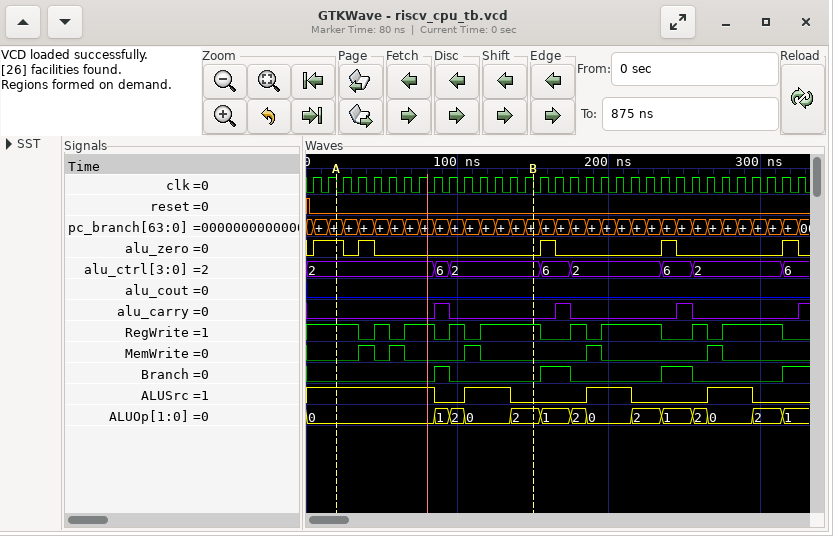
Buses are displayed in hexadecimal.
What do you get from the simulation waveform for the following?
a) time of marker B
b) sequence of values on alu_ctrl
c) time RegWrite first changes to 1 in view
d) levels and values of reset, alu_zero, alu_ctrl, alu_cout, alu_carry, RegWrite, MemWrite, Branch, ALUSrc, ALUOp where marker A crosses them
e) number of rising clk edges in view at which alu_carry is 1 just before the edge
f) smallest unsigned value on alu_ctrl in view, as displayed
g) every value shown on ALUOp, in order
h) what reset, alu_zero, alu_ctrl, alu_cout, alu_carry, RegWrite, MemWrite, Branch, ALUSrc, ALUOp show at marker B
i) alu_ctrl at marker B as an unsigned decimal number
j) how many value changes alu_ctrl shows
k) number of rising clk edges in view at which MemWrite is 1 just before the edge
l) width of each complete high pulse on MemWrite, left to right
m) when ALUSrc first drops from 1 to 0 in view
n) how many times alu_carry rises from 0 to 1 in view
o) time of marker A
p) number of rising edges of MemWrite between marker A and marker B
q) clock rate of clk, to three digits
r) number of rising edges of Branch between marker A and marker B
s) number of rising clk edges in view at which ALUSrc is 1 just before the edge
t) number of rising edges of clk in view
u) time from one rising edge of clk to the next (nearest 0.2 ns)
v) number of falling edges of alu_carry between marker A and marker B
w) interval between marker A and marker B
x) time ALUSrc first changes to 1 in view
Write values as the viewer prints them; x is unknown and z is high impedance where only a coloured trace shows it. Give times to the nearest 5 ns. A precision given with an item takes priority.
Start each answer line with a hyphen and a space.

- 150 ns
- 2, 6, 2, 6, 2, 6, 2, 6
- 45 ns
- reset=0, alu_zero=1, alu_ctrl=2, alu_cout=0, alu_carry=0, RegWrite=1, MemWrite=0, Branch=0, ALUSrc=1, ALUOp=0
- 3
- 2
- 0, 1, 2, 0, 2, 1, 2, 0, 2, 1, 2, 0, 2, 1
- reset=0, alu_zero=0, alu_ctrl=2, alu_cout=0, alu_carry=0, RegWrite=1, MemWrite=0, Branch=0, ALUSrc=0, ALUOp=2
- 2
- 7
- 5
- 10 ns, 10 ns, 10 ns, 10 ns, 10 ns
- 85 ns
- 4
- 20 ns
- 3
- 100 MHz
- 1
- 18
- 33
- 10 ns
- 1
- 130 ns
- 105 ns
